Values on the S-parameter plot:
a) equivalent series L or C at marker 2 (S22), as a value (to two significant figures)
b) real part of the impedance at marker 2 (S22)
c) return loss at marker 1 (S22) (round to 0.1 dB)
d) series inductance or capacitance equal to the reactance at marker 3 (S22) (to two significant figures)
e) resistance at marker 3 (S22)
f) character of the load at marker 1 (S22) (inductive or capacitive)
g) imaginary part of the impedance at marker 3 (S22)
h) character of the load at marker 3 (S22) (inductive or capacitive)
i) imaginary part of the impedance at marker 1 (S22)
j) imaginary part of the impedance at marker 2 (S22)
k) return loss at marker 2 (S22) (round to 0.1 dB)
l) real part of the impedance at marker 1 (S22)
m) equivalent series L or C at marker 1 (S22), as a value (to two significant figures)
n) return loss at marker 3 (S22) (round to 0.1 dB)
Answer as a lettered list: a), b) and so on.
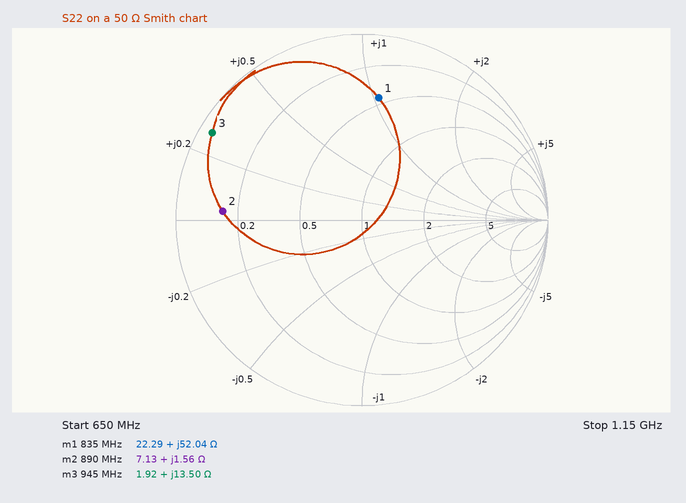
a) 280 pH
b) 7.13 Ω
c) 3.6 dB
d) 2.3 nH
e) 1.92 Ω
f) inductive
g) +13.50 Ω
h) inductive
i) +52.04 Ω
j) +1.56 Ω
k) 2.5 dB
l) 22.29 Ω
m) 9.9 nH
n) 0.6 dB
